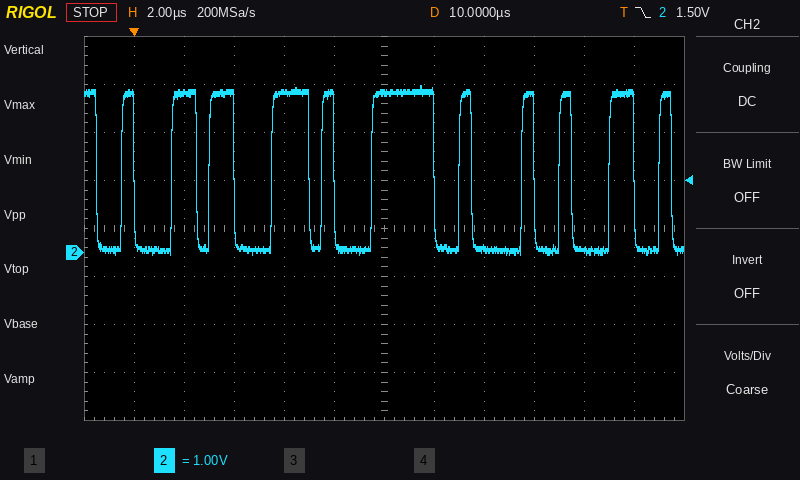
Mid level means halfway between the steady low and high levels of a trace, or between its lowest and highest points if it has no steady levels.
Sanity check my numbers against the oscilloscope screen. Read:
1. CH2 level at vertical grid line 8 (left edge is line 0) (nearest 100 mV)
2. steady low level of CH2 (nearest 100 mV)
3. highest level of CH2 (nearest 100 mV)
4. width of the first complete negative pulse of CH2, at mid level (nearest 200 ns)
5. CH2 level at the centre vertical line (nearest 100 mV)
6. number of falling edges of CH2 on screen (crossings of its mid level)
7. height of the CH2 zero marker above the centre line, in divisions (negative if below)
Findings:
100 mV
100 mV
3.5 V
1.0 µs
3.3 V
12
-0.5 div
